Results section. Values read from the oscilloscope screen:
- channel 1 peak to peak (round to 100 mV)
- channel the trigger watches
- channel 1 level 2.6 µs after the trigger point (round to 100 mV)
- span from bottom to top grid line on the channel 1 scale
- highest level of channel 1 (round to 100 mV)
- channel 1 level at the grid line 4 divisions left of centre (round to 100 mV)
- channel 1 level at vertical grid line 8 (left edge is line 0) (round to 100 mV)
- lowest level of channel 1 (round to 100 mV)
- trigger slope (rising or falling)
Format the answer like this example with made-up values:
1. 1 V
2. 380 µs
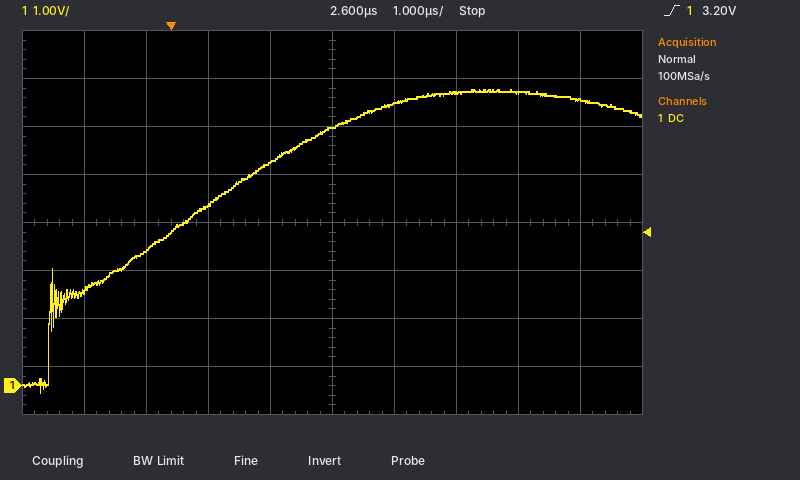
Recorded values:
1. 6.3 V
2. channel 1
3. 5.4 V
4. 8 V
5. 6.2 V
6. 2.0 V
7. 6.1 V
8. -100 mV
9. rising
